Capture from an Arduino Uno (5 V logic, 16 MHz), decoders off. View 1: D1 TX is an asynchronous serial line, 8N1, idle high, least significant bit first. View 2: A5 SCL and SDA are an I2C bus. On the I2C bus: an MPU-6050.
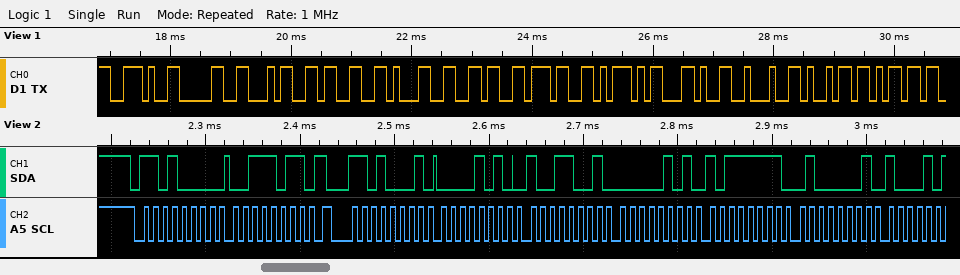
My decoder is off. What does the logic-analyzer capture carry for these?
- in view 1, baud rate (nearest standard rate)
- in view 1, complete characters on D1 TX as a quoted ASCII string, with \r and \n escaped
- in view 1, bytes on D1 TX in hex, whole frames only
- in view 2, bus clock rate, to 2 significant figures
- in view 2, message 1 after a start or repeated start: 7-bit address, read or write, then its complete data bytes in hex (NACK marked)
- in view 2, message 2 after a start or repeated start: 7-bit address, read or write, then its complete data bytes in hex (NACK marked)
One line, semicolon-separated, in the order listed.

9600 baud; ".043167],\"im"; 2E 30 34 33 31 36 37 5D 2C 22 69 6D; 100 kHz; 0x68 write: 3B; 0x68 read: 0A 99 05 BF 41
